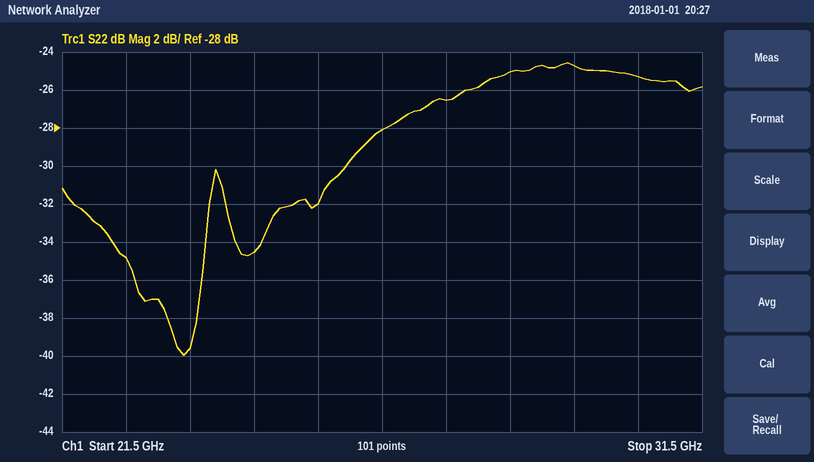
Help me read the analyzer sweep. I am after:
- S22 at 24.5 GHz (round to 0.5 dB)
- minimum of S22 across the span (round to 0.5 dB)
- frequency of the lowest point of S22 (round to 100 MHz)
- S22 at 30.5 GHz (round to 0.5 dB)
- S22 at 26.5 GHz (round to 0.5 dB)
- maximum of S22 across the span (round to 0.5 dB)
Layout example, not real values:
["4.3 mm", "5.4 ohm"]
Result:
["-34.5 dB", "-40.0 dB", "23.4 GHz", "-25.5 dB", "-28.0 dB", "-24.5 dB"]
